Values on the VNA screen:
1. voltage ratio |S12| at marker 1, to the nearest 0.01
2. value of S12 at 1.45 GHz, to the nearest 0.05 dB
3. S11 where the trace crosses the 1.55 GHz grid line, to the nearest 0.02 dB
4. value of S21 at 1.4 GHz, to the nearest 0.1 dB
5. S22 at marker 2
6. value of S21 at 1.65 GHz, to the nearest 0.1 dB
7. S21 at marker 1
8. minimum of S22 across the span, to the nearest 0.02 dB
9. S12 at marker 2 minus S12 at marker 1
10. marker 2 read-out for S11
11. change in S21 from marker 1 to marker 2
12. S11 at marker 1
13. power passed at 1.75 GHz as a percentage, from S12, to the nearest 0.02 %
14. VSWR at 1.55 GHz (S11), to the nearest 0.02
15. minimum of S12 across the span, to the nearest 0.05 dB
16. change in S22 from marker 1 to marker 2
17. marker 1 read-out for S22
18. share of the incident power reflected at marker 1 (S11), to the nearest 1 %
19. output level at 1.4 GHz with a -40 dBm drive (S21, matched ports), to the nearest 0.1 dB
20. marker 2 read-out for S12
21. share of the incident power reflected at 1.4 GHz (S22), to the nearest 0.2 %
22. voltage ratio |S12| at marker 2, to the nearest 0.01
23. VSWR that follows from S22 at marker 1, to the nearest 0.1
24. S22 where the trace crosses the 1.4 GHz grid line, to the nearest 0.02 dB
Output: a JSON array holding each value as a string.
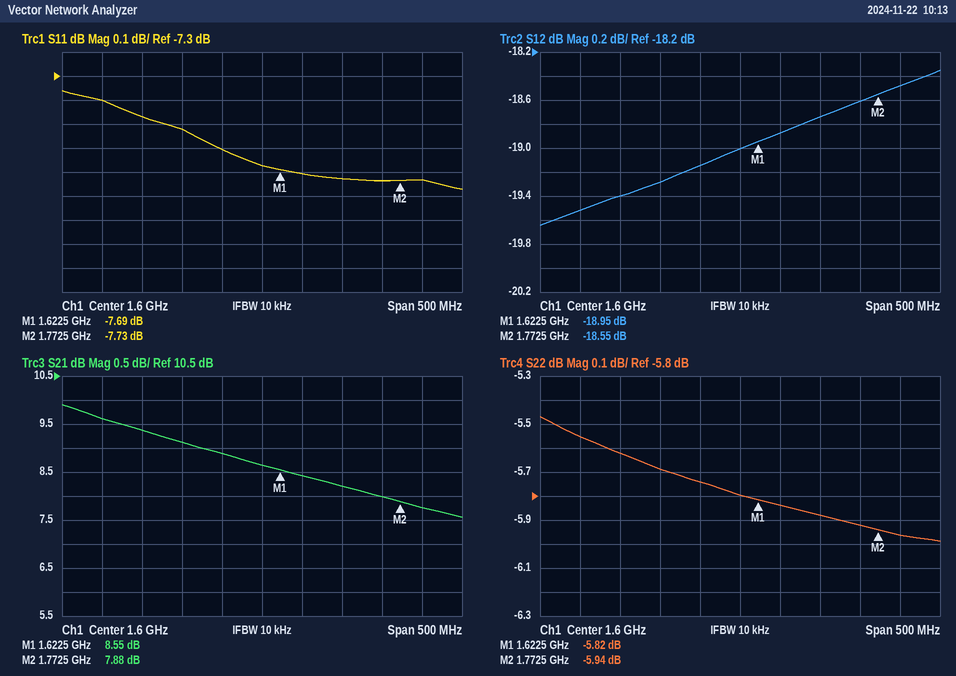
["0.11", "-19.40 dB", "-7.60 dB", "9.6 dB", "-5.94 dB", "8.4 dB", "8.55 dB", "-5.98 dB", "0.40 dB", "-7.73 dB", "-0.67 dB", "-7.69 dB", "1.38 %", "2.42", "-19.65 dB", "-0.12 dB", "-5.82 dB", "17 %", "-30.4 dBm", "-18.55 dB", "27.8 %", "0.12", "3.1", "-5.56 dB"]
